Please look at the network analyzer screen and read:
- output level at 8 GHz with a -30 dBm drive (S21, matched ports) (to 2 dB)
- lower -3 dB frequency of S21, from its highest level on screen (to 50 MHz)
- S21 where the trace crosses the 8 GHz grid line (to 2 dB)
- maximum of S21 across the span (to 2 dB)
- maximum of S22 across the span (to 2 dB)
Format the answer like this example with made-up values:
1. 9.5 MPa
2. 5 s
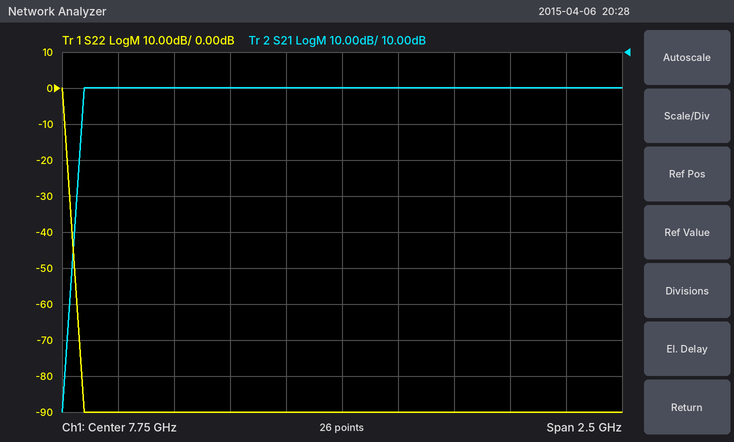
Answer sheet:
1. -30 dBm
2. 6.60 GHz
3. 0 dB
4. 0 dB
5. 0 dB
